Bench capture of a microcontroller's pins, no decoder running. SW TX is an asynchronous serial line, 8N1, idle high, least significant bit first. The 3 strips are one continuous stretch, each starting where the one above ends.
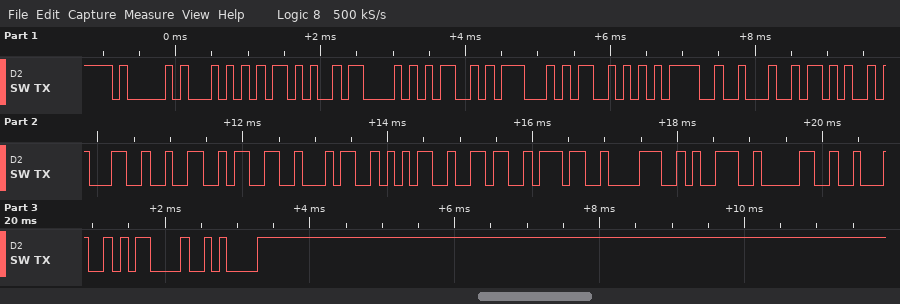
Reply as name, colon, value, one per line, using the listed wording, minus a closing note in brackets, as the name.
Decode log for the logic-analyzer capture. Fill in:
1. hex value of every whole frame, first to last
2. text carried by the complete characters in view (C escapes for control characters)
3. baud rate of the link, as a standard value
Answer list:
hex value of every whole frame, first to last: 41 54 2B 43 4D 47 53 3D 22 2B 31 32 33 34 35 36 37 38 39 30 22 0D 0A
text carried by the complete characters in view: "AT+CMGS=\"+1234567890\"\r\n"
baud rate of the link, as a standard value: 9600 baud
